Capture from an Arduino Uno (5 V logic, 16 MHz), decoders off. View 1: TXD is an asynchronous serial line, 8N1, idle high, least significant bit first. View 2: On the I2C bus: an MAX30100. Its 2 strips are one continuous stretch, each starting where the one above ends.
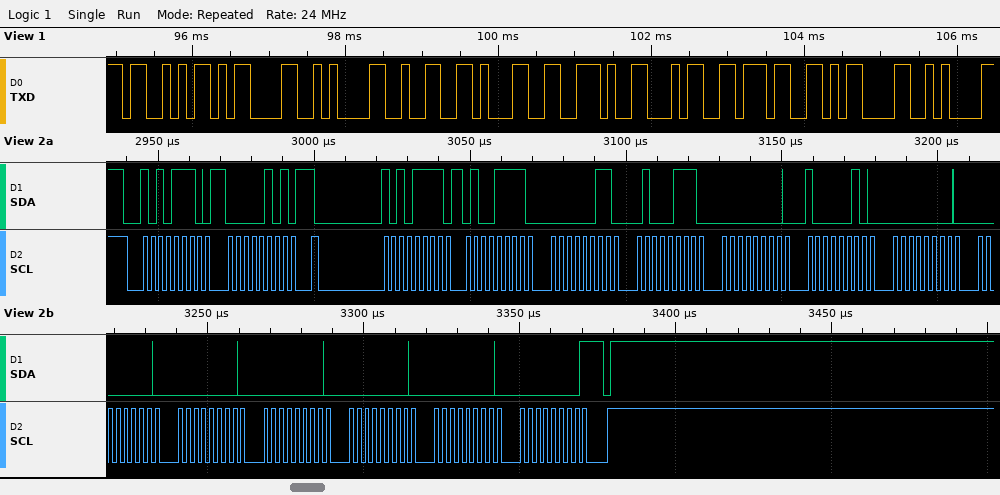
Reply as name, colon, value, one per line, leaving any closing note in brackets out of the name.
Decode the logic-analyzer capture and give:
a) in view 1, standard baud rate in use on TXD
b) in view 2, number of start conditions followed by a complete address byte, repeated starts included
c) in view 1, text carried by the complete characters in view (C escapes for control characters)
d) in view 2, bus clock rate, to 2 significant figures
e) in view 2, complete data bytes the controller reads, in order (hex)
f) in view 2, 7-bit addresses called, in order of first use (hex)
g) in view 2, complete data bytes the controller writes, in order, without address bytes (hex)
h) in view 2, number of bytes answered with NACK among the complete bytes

in view 1, standard baud rate in use on TXD: 9600 baud
in view 2, number of start conditions followed by a complete address byte, repeated starts included: 2
in view 1, text carried by the complete characters in view: "S\r\n21.47\r\n"
in view 2, bus clock rate, to 2 significant figures: 400 kHz
in view 2, complete data bytes the controller reads, in order: 4F 03 47 00 82 00 00 00 00 00 00 00
in view 2, 7-bit addresses called, in order of first use: 0x57
in view 2, complete data bytes the controller writes, in order, without address bytes: 05
in view 2, number of bytes answered with NACK among the complete bytes: 1
